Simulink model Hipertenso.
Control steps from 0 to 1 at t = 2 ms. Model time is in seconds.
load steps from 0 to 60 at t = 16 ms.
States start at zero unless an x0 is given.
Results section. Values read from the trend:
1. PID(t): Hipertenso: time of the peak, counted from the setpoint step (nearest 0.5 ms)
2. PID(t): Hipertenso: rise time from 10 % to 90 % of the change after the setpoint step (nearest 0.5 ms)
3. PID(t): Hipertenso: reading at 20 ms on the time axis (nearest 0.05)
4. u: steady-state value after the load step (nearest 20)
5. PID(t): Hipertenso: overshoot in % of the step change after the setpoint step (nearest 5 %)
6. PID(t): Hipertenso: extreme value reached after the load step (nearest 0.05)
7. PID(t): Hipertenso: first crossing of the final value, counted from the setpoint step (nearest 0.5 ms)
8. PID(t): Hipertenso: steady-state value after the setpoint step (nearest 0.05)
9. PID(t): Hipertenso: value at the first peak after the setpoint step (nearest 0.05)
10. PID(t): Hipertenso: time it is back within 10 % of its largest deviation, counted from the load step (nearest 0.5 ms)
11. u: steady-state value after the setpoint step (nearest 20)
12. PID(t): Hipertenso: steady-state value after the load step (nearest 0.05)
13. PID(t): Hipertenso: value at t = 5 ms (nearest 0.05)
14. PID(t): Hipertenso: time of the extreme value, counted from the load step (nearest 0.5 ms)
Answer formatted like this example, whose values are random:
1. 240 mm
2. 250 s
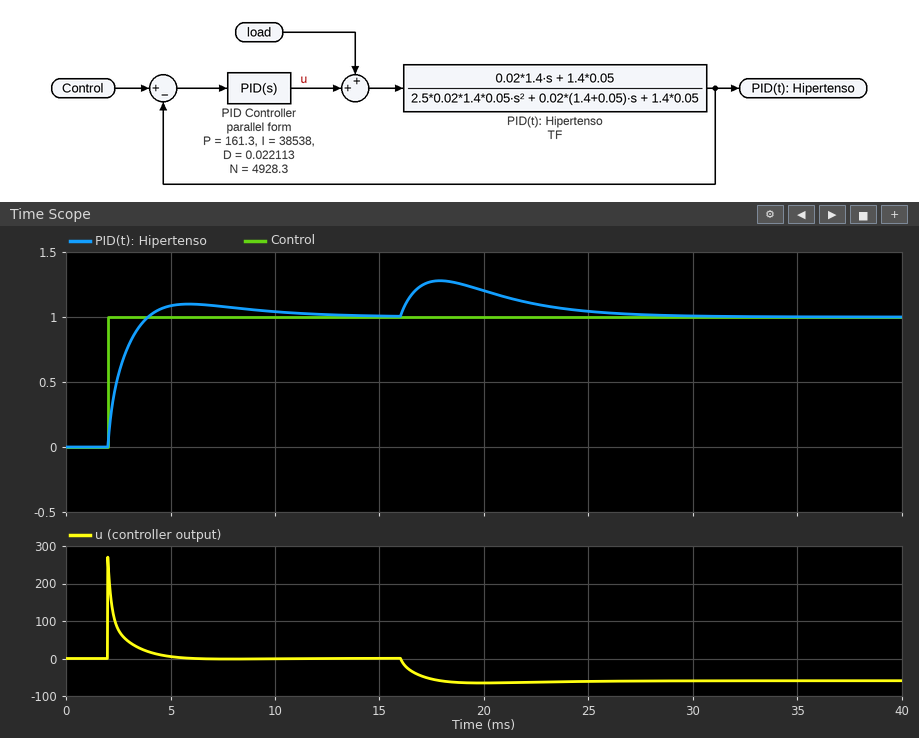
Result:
1. 4.0 ms
2. 1.5 ms
3. 1.20
4. -60
5. 10 %
6. 1.30
7. 2.0 ms
8. 1.00
9. 1.10
10. 10.5 ms
11. 0
12. 1.00
13. 1.10
14. 2.0 ms
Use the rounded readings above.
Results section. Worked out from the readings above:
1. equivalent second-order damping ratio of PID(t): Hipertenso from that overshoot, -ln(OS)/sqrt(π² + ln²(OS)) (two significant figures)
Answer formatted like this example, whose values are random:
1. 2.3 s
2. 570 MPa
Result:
1. 0.59
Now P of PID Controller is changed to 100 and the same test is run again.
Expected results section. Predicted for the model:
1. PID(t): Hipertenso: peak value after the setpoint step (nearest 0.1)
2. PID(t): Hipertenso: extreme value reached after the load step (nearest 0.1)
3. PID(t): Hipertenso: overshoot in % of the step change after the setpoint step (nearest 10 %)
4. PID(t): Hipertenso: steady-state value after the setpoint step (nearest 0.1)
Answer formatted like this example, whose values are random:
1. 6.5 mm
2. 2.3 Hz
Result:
1. 1.2
2. 1.4
3. 20 %
4. 1.0
